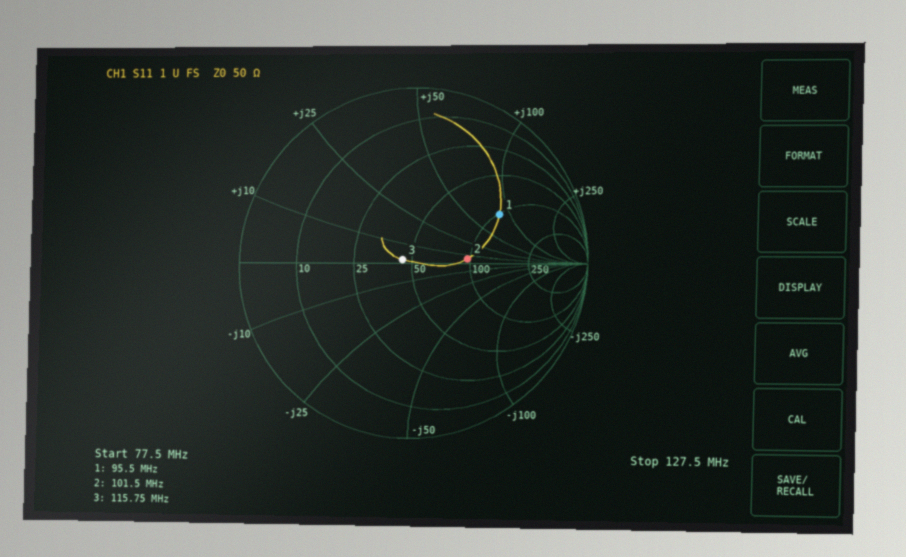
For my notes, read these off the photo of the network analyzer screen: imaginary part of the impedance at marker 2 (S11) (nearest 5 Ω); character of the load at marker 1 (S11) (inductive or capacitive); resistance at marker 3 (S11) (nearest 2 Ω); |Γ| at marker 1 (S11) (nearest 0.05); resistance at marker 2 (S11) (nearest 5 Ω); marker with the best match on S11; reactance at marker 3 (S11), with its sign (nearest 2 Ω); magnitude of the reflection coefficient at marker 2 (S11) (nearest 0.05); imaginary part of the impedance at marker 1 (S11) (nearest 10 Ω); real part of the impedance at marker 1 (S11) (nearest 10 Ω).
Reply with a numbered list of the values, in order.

1. +5 Ω
2. inductive
3. 44 Ω
4. 0.55
5. 95 Ω
6. marker 3
7. +2 Ω
8. 0.30
9. +80 Ω
10. 100 Ω
